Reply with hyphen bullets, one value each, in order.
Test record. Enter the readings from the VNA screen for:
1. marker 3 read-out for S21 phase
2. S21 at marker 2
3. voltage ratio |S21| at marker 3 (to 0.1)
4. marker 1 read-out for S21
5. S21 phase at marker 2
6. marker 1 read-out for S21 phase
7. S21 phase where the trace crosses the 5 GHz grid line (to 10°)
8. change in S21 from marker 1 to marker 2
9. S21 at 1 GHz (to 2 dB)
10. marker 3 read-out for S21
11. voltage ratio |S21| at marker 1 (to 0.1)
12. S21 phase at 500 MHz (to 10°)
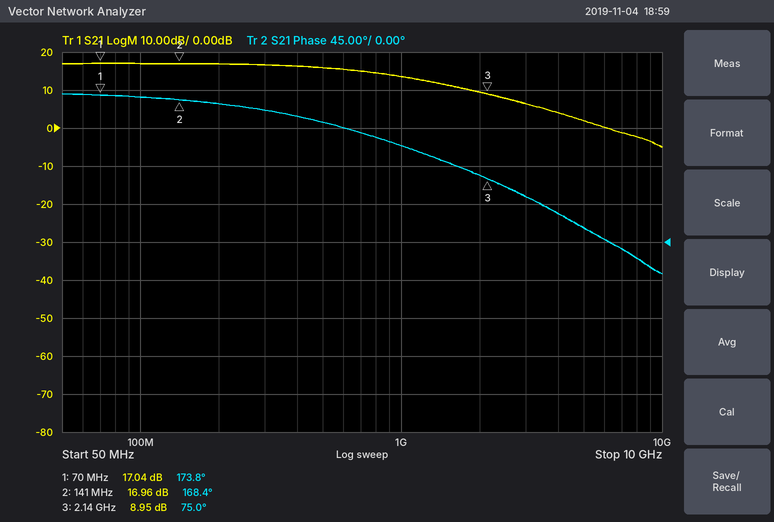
- 75.0°
- 16.96 dB
- 2.8
- 17.04 dB
- 168.4°
- 173.8°
- 20°
- -0.08 dB
- 14 dB
- 8.95 dB
- 7.1
- 140°
